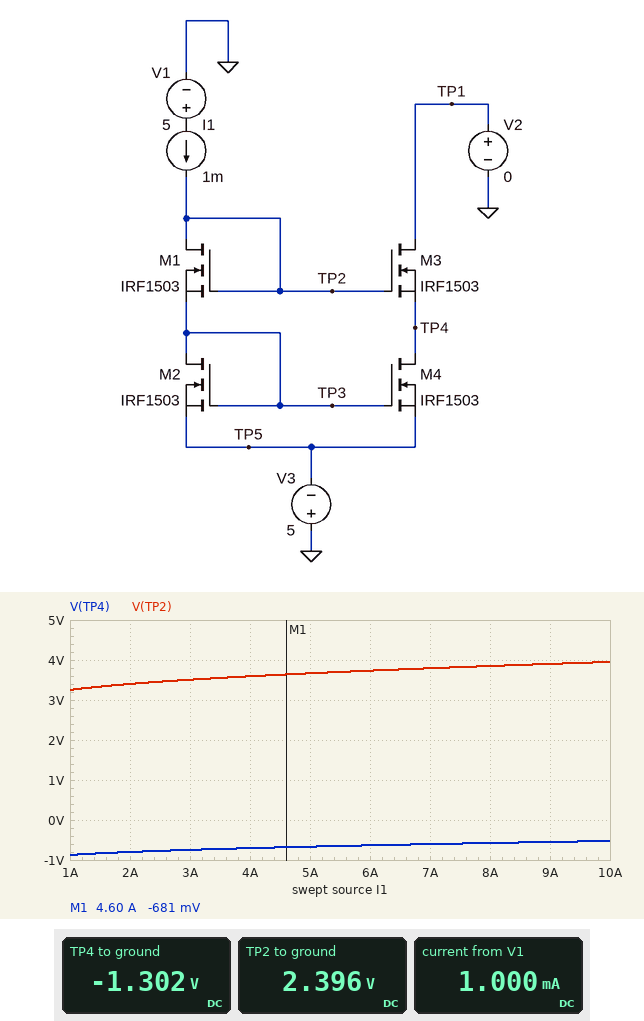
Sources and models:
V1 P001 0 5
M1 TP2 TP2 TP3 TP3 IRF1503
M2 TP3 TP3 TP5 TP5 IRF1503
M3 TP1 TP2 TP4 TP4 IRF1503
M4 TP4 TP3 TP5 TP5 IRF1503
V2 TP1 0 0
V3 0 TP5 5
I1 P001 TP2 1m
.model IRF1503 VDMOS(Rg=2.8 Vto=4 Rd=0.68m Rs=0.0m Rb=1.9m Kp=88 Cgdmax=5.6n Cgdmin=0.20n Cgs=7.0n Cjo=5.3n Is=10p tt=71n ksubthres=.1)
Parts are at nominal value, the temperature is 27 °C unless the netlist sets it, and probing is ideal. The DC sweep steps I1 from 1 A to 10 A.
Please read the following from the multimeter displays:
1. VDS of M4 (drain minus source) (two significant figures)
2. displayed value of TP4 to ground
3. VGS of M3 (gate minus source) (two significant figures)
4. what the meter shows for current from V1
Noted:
3.7 V
-1.302 V
3.7 V
1.000 mA
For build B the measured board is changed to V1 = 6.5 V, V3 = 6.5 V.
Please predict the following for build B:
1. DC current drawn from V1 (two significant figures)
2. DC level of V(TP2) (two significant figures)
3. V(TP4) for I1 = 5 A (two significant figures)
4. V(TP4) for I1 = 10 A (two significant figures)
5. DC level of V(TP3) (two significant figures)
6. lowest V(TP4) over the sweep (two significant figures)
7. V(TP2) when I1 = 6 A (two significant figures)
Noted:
1.0 mA
900 mV
-2.2 V
-2.0 V
-2.8 V
-2.4 V
2.2 V
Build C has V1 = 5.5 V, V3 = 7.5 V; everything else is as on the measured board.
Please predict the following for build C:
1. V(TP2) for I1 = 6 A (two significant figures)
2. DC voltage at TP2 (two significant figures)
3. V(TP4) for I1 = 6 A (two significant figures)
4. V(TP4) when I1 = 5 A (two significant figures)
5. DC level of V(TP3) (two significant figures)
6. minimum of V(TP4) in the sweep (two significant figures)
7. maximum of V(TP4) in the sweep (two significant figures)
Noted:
1.2 V
-100 mV
-3.1 V
-3.2 V
-3.8 V
-3.4 V
-3.0 V
